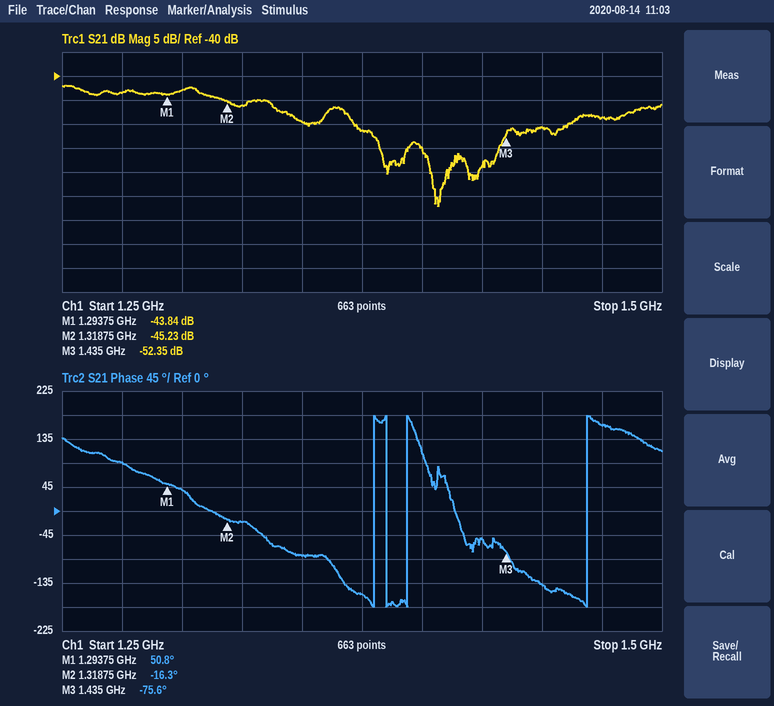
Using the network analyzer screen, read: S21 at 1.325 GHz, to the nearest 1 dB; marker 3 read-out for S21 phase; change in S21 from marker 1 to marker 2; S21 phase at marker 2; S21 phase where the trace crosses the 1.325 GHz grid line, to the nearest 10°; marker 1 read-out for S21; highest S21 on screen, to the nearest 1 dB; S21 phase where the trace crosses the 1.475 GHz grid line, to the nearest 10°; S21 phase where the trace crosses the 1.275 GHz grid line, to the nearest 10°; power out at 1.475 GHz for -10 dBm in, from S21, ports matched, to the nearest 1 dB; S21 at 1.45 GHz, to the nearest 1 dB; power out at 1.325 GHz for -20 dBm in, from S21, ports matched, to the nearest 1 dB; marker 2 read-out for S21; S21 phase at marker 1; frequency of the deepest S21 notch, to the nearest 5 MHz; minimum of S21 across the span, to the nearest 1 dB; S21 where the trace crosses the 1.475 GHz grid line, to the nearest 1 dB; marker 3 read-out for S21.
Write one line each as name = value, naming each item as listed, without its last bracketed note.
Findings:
S21 at 1.325 GHz, to the nearest 1 dB = -46 dB
marker 3 read-out for S21 phase = -75.6°
change in S21 from marker 1 to marker 2 = -1.39 dB
S21 phase at marker 2 = -16.3°
S21 phase where the trace crosses the 1.325 GHz grid line, to the nearest 10° = -20°
marker 1 read-out for S21 = -43.84 dB
highest S21 on screen, to the nearest 1 dB = -42 dB
S21 phase where the trace crosses the 1.475 GHz grid line, to the nearest 10° = 160°
S21 phase where the trace crosses the 1.275 GHz grid line, to the nearest 10° = 90°
power out at 1.475 GHz for -10 dBm in, from S21, ports matched, to the nearest 1 dB = -59 dBm
S21 at 1.45 GHz, to the nearest 1 dB = -51 dB
power out at 1.325 GHz for -20 dBm in, from S21, ports matched, to the nearest 1 dB = -66 dBm
marker 2 read-out for S21 = -45.23 dB
S21 phase at marker 1 = 50.8°
frequency of the deepest S21 notch, to the nearest 5 MHz = 1.405 GHz
minimum of S21 across the span, to the nearest 1 dB = -67 dB
S21 where the trace crosses the 1.475 GHz grid line, to the nearest 1 dB = -49 dB
marker 3 read-out for S21 = -52.35 dB
